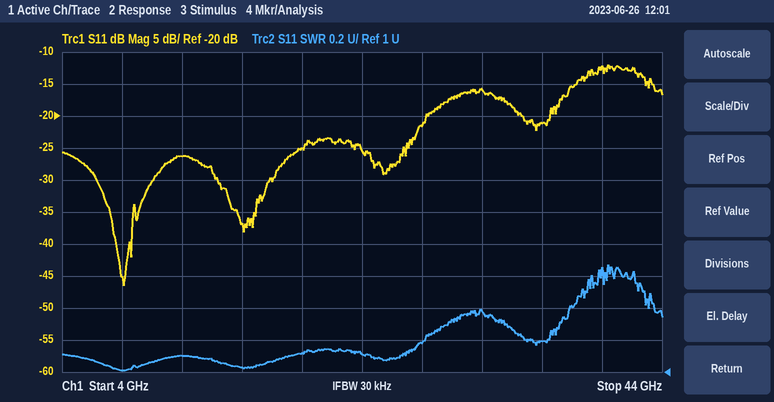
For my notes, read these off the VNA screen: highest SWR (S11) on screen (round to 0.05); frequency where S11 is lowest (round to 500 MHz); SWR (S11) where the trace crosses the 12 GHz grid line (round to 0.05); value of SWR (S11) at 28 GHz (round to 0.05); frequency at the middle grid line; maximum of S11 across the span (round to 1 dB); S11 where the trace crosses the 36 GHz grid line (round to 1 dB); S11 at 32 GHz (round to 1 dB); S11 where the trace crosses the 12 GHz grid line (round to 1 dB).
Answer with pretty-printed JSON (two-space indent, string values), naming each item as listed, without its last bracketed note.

{
  "highest SWR (S11) on screen": "1.65",
  "frequency where S11 is lowest": "8.0 GHz",
  "SWR (S11) where the trace crosses the 12 GHz grid line": "1.10",
  "value of SWR (S11) at 28 GHz": "1.20",
  "frequency at the middle grid line": "24 GHz",
  "maximum of S11 across the span": "-12 dB",
  "S11 where the trace crosses the 36 GHz grid line": "-21 dB",
  "S11 at 32 GHz": "-16 dB",
  "S11 where the trace crosses the 12 GHz grid line": "-26 dB"
}
